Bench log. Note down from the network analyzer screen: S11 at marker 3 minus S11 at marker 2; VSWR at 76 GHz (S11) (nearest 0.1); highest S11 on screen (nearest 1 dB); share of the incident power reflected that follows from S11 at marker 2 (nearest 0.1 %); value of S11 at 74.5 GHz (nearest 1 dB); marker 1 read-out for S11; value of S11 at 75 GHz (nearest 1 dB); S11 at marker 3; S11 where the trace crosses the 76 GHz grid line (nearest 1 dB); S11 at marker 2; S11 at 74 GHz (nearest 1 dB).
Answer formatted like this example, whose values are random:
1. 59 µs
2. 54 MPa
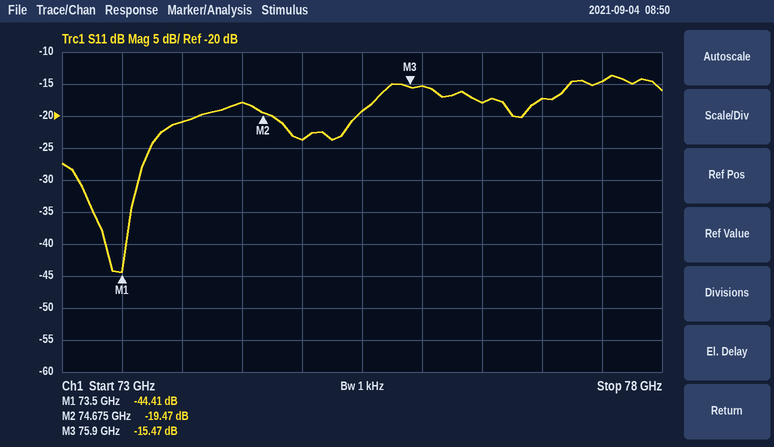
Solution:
1. 4.00 dB
2. 1.4
3. -14 dB
4. 1.1 %
5. -18 dB
6. -44.41 dB
7. -24 dB
8. -15.47 dB
9. -15 dB
10. -19.47 dB
11. -21 dB
